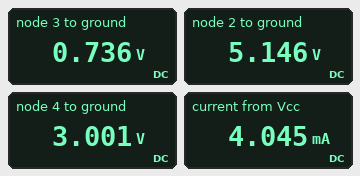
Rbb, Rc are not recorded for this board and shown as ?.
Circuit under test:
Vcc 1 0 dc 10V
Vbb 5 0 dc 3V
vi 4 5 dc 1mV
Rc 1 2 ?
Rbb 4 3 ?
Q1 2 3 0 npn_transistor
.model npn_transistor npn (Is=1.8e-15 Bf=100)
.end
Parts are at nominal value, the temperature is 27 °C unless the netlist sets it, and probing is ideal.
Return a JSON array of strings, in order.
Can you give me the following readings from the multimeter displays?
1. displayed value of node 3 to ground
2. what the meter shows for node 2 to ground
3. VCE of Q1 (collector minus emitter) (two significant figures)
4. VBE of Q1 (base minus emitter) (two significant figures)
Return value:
["0.736 V", "5.146 V", "5.1 V", "740 mV"]
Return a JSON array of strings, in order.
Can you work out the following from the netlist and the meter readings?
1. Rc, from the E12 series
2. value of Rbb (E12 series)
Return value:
["1.2 kΩ", "56 kΩ"]
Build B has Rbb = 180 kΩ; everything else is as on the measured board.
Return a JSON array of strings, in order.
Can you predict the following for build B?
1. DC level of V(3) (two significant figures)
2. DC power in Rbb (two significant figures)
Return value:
["710 mV", "29 µW"]
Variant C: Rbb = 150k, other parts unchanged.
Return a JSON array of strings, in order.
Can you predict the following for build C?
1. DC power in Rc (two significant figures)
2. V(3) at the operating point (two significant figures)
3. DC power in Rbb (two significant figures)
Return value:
["2.8 mW", "710 mV", "35 µW"]
